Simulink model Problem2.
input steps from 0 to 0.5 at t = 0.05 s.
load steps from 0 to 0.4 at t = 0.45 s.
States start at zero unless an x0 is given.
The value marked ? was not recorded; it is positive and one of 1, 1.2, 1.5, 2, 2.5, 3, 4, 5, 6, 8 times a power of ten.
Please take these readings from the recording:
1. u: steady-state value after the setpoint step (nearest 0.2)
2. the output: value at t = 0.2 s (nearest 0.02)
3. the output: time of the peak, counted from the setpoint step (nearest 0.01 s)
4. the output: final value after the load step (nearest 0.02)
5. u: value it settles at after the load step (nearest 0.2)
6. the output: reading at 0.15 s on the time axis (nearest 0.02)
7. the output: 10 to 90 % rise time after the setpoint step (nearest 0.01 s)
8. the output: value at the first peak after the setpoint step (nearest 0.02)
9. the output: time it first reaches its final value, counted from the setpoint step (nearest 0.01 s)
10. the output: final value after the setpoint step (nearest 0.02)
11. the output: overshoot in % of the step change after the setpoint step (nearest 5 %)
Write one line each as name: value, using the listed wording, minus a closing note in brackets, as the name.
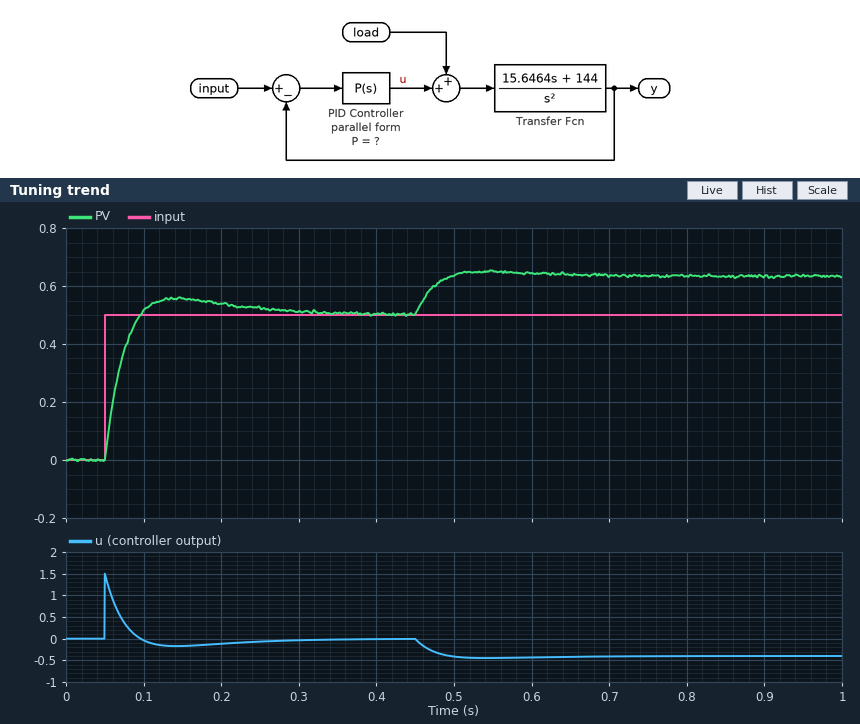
u: steady-state value after the setpoint step: 0.0
the output: value at t = 0.2 s: 0.54
the output: time of the peak, counted from the setpoint step: 0.09 s
the output: final value after the load step: 0.64
u: value it settles at after the load step: -0.4
the output: reading at 0.15 s on the time axis: 0.56
the output: 10 to 90 % rise time after the setpoint step: 0.03 s
the output: value at the first peak after the setpoint step: 0.56
the output: time it first reaches its final value, counted from the setpoint step: 0.05 s
the output: final value after the setpoint step: 0.50
the output: overshoot in % of the step change after the setpoint step: 10 %
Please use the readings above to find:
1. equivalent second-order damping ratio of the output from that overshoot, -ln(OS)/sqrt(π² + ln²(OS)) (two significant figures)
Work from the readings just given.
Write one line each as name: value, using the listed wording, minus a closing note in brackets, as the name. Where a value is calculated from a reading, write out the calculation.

equivalent second-order damping ratio of the output from that overshoot, -ln(OS)/sqrt(π² + ln²(OS)): ln(0.1) = -2.303; 2.303 / sqrt(9.870 + 5.302) = 0.59
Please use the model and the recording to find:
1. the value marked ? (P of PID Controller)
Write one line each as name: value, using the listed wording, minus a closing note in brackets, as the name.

the value marked ?: 3
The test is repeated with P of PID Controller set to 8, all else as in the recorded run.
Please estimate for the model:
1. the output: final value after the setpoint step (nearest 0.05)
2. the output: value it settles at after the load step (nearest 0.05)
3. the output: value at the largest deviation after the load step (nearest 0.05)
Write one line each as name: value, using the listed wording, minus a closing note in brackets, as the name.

the output: final value after the setpoint step: 0.50
the output: value it settles at after the load step: 0.55
the output: value at the largest deviation after the load step: 0.55
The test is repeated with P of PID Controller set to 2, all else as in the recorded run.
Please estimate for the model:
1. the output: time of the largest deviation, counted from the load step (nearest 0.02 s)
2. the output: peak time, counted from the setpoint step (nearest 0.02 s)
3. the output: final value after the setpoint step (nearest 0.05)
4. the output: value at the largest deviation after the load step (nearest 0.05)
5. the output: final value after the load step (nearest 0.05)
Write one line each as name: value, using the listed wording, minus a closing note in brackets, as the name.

the output: time of the largest deviation, counted from the load step: 0.12 s
the output: peak time, counted from the setpoint step: 0.12 s
the output: final value after the setpoint step: 0.50
the output: value at the largest deviation after the load step: 0.75
the output: final value after the load step: 0.70
